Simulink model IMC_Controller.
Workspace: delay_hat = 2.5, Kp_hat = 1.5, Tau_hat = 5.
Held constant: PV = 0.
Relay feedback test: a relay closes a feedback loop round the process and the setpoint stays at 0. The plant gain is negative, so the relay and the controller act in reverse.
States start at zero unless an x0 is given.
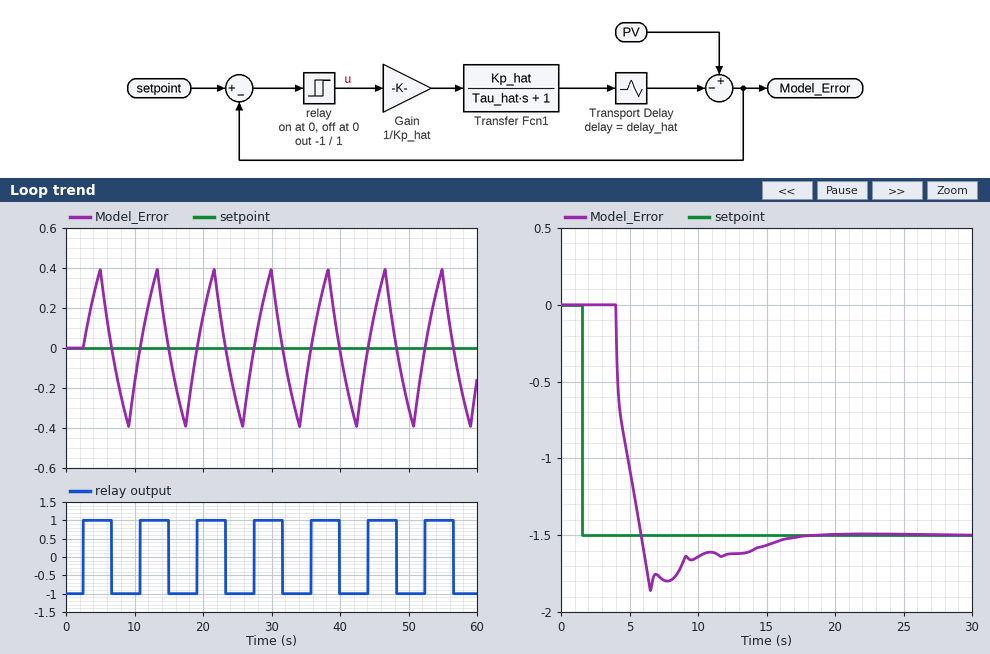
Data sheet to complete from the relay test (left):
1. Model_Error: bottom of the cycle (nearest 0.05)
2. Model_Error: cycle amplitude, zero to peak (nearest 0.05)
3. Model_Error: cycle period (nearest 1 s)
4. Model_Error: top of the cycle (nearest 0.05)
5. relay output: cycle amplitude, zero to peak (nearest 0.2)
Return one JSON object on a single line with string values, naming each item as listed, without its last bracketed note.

{"Model_Error: bottom of the cycle": "-0.40", "Model_Error: cycle amplitude, zero to peak": "0.40", "Model_Error: cycle period": "8 s", "Model_Error: top of the cycle": "0.40", "relay output: cycle amplitude, zero to peak": "1.0"}
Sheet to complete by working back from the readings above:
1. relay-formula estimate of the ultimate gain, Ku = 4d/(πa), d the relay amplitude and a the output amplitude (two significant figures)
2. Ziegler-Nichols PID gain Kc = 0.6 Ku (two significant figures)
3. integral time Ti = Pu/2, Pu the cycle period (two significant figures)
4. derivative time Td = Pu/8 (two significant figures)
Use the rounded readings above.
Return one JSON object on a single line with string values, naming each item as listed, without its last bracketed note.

{"relay-formula estimate of the ultimate gain, Ku = 4d/(πa), d the relay amplitude and a the output amplitude": "3.2", "Ziegler-Nichols PID gain Kc = 0.6 Ku": "1.9", "integral time Ti = Pu/2, Pu the cycle period": "4.0 s", "derivative time Td = Pu/8": "1.0 s"}
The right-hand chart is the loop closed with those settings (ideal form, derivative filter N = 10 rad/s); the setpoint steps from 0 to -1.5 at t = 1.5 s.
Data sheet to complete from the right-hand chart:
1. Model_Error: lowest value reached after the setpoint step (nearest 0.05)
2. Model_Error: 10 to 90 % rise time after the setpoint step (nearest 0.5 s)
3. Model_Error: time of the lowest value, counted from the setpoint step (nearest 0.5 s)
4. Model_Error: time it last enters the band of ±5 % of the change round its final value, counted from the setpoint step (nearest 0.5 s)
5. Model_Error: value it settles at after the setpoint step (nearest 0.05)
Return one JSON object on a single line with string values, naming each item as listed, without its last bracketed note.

{"Model_Error: lowest value reached after the setpoint step": "-1.85", "Model_Error: 10 to 90 % rise time after the setpoint step": "1.5 s", "Model_Error: time of the lowest value, counted from the setpoint step": "5.0 s", "Model_Error: time it last enters the band of ±5 % of the change round its final value, counted from the setpoint step": "13.0 s", "Model_Error: value it settles at after the setpoint step": "-1.50"}
